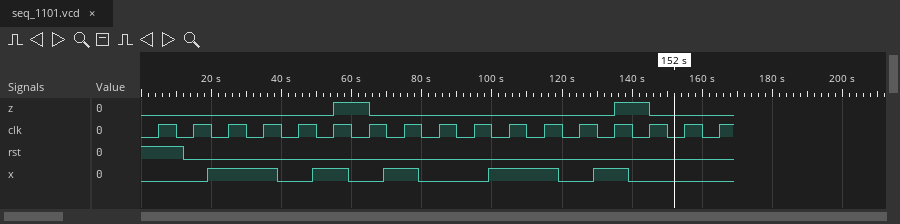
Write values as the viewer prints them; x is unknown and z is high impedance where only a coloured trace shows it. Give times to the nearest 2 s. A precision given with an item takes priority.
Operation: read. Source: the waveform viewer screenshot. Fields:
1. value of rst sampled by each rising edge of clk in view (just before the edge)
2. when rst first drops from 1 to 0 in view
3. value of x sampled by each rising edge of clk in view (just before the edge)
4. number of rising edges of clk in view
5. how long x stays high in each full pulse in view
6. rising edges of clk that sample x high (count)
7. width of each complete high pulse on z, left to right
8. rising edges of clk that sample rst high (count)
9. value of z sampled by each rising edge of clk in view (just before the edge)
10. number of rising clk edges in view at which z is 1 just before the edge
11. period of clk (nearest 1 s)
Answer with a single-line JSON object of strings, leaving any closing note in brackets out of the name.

{"value of rst sampled by each rising edge of clk in view": "1 0 0 0 0 0 0 0 0 0 0 0 0 0 0 0 0", "when rst first drops from 1 to 0 in view": "12 s", "value of x sampled by each rising edge of clk in view": "0 0 1 1 0 1 0 1 0 0 1 1 0 1 0 0 0", "number of rising edges of clk in view": "17", "how long x stays high in each full pulse in view": "20 s, 10 s, 10 s, 20 s, 10 s", "rising edges of clk that sample x high": "7", "width of each complete high pulse on z, left to right": "10 s, 10 s", "rising edges of clk that sample rst high": "1", "value of z sampled by each rising edge of clk in view": "0 0 0 0 0 0 1 0 0 0 0 0 0 0 1 0 0", "number of rising clk edges in view at which z is 1 just before the edge": "2", "period of clk": "10 s"}
